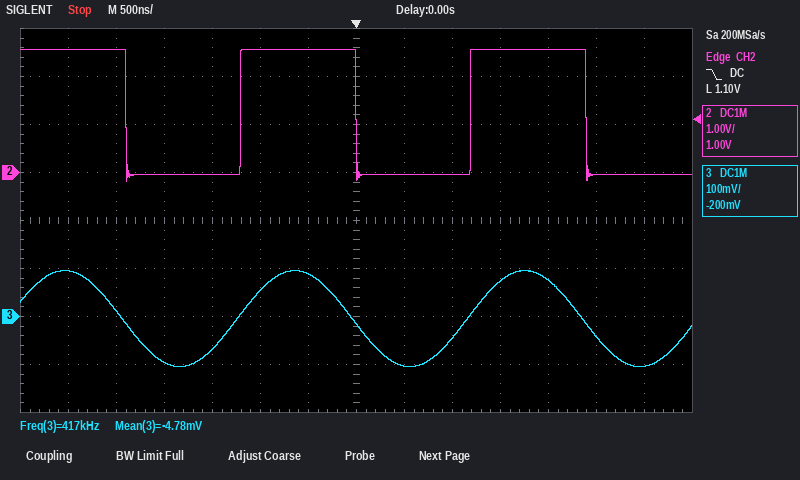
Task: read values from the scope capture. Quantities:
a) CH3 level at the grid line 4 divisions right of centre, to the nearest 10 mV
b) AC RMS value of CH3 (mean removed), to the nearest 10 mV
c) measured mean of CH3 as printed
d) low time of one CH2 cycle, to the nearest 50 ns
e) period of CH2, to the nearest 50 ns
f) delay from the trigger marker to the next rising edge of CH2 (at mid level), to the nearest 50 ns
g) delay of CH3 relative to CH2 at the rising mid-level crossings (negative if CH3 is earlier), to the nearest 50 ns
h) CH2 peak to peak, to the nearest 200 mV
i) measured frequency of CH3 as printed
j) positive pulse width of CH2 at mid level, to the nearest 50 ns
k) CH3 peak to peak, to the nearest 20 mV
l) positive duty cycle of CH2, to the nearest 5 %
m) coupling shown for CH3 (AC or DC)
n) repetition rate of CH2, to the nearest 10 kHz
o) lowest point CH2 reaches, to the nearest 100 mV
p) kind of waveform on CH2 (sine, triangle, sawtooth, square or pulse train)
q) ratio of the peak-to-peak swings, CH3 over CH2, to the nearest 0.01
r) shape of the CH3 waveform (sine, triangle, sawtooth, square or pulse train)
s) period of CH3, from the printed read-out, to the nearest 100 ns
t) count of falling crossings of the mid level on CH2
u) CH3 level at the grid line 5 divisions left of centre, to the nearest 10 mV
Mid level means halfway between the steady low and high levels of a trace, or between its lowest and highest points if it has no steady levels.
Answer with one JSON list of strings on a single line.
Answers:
["80 mV", "70 mV", "-4.78 mV", "1.20 µs", "2.40 µs", "1.20 µs", "-50 ns", "2.8 V", "417 kHz", "1.20 µs", "200 mV", "50 %", "DC", "420 kHz", "-200 mV", "square", "0.07", "sine", "2.4 µs", "3", "10 mV"]
